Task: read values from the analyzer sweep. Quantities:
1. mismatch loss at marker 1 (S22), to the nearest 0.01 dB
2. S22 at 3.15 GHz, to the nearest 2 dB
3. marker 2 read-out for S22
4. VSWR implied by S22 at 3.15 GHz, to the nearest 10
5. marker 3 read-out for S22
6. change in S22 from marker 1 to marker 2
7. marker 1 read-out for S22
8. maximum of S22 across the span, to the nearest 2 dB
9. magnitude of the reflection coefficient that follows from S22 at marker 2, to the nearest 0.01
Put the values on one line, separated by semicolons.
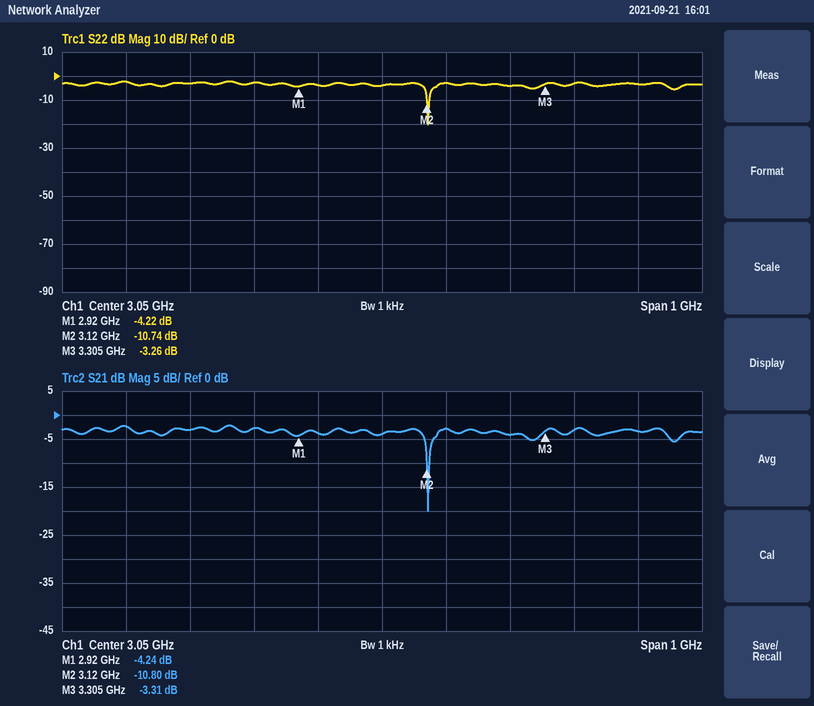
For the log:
2.07 dB; -2 dB; -10.74 dB; 10; -3.26 dB; -6.52 dB; -4.22 dB; -2 dB; 0.29
